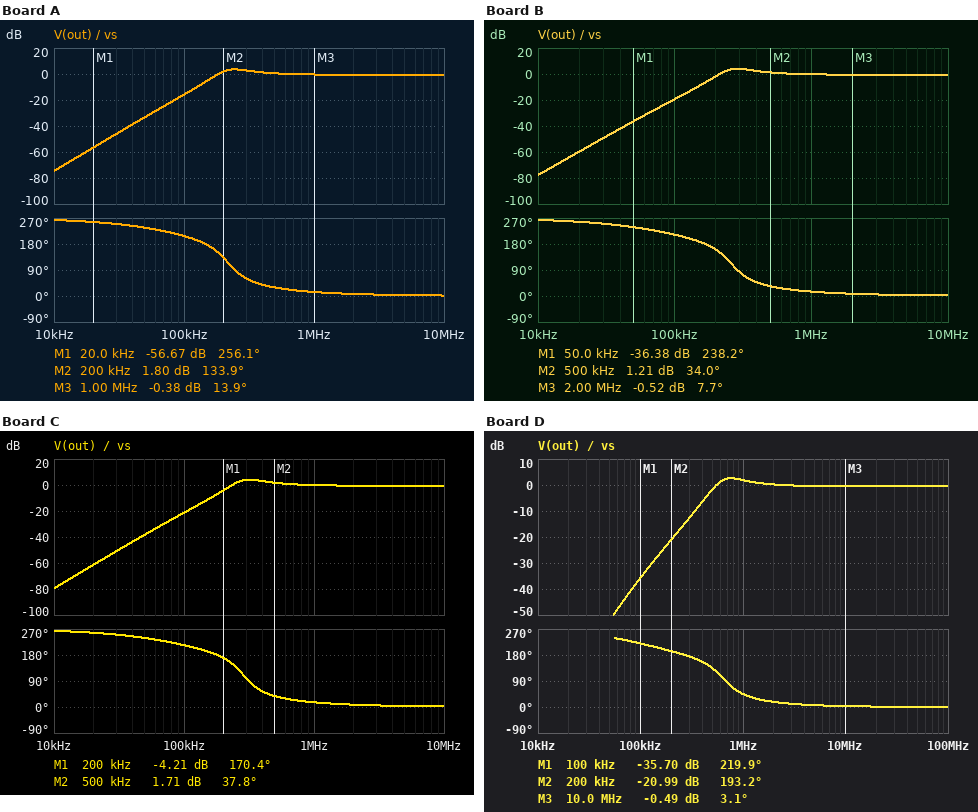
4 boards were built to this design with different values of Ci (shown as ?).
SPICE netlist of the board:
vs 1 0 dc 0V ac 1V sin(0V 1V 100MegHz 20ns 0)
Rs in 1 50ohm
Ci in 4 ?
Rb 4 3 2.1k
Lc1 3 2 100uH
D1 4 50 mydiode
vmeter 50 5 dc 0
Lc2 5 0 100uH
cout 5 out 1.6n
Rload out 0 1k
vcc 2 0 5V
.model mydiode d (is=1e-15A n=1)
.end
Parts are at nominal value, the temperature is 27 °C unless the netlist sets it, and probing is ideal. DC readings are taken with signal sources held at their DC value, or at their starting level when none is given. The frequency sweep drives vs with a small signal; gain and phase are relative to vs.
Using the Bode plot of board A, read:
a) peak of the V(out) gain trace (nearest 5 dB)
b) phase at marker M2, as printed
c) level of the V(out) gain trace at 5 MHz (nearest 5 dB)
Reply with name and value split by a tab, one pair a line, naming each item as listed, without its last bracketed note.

peak of the V(out) gain trace	5 dB
phase at marker M2, as printed	133.9 deg
level of the V(out) gain trace at 5 MHz	0 dB
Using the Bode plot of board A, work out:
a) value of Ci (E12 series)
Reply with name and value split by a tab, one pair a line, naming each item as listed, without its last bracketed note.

value of Ci	4.7 nF
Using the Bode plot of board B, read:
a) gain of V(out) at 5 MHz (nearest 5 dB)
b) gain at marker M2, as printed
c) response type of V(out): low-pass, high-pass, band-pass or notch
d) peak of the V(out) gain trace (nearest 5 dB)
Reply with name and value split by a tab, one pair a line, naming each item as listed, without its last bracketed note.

gain of V(out) at 5 MHz	0 dB
gain at marker M2, as printed	1.21 dB
response type of V(out): low-pass, high-pass, band-pass or notch	high-pass
peak of the V(out) gain trace	5 dB
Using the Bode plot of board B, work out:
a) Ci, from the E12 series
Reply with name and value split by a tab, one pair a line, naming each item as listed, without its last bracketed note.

Ci, from the E12 series	3.3 nF
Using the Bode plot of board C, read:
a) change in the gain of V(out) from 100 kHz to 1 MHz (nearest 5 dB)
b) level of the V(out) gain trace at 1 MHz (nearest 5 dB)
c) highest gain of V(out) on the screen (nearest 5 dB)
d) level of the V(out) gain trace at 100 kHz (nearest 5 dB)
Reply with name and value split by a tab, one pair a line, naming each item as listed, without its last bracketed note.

change in the gain of V(out) from 100 kHz to 1 MHz	20 dB
level of the V(out) gain trace at 1 MHz	0 dB
highest gain of V(out) on the screen	5 dB
level of the V(out) gain trace at 100 kHz	-20 dB
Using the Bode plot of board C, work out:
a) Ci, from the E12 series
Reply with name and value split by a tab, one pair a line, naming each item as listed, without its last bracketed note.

Ci, from the E12 series	2.7 nF
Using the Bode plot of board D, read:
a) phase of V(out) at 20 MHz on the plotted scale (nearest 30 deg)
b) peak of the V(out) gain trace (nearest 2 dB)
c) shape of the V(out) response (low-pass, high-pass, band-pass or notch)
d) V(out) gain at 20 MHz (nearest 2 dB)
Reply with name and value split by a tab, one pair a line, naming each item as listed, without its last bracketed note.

phase of V(out) at 20 MHz on the plotted scale	0 deg
peak of the V(out) gain trace	2 dB
shape of the V(out) response	high-pass
V(out) gain at 20 MHz	0 dB
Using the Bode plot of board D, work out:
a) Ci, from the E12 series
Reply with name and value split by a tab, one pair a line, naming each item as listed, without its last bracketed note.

Ci, from the E12 series	560 pF
